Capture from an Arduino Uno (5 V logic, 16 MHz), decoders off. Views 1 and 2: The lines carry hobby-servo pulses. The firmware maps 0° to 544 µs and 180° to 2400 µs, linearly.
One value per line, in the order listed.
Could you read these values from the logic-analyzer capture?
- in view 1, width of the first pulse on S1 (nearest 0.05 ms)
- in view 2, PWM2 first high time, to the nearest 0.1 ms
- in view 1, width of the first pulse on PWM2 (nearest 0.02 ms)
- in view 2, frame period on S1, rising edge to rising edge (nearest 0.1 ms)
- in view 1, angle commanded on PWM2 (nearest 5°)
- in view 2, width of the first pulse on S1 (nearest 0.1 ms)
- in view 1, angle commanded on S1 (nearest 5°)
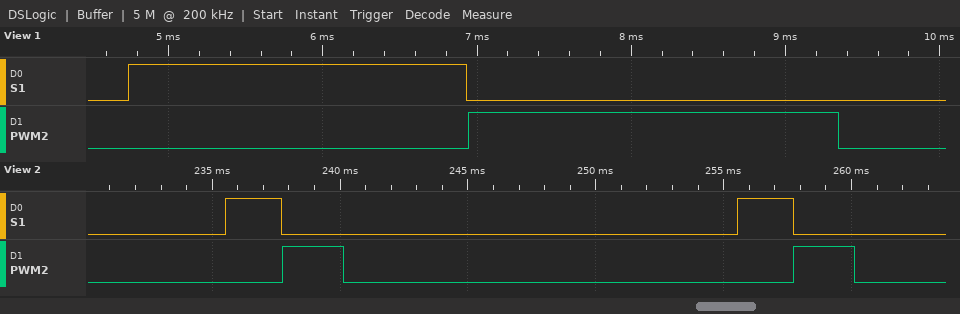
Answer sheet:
2.20 ms
2.4 ms
2.40 ms
20.0 ms
180°
2.2 ms
160°
